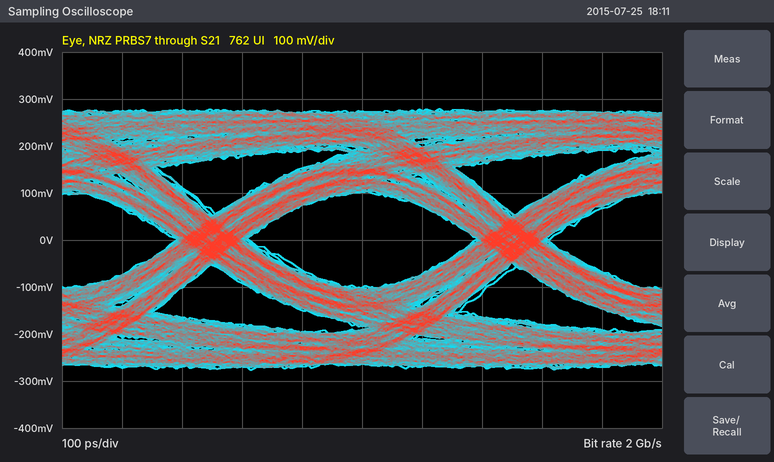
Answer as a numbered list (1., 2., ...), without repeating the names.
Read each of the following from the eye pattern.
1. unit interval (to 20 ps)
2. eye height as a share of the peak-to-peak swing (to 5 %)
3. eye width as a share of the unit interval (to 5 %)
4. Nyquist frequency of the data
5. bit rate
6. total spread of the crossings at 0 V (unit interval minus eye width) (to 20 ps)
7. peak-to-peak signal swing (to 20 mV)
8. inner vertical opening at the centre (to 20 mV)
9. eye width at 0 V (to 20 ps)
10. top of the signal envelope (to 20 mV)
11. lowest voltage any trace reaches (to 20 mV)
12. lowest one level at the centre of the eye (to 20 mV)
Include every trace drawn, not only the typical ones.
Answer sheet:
1. 500 ps
2. 35 %
3. 75 %
4. 1 GHz
5. 2 Gb/s
6. 120 ps
7. 560 mV
8. 200 mV
9. 380 ps
10. 280 mV
11. -280 mV
12. 100 mV
